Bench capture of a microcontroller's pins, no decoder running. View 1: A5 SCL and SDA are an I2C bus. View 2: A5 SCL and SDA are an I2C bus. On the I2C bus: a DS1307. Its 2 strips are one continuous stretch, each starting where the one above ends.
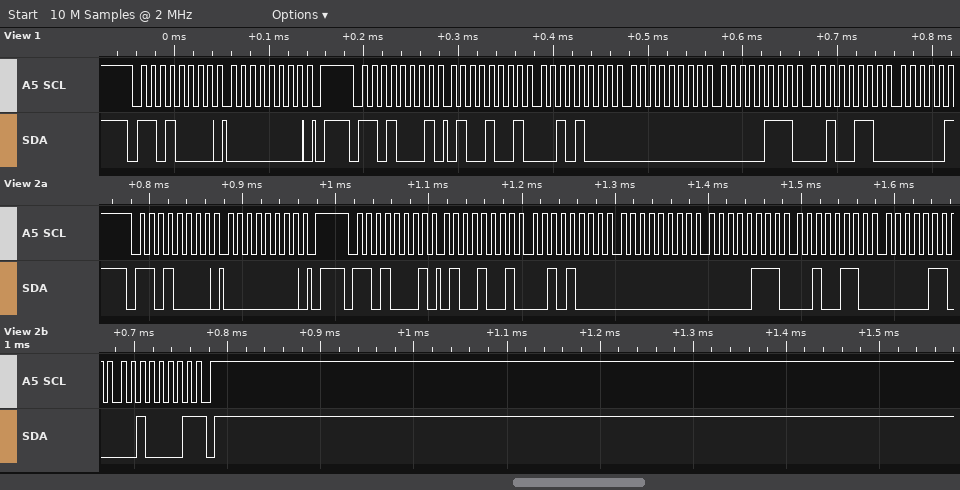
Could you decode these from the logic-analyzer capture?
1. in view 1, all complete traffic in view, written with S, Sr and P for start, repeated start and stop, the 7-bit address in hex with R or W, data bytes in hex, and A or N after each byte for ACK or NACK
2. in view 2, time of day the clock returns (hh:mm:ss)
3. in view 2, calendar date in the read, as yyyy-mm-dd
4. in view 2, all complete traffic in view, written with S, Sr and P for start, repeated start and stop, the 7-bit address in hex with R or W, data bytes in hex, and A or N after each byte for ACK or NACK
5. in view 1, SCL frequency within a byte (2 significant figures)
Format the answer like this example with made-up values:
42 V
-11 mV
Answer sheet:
S 68W A 00 A P S 68R A 49 A 28 A 00 A 07 A 26 A
00:28:49
2021-06-26
S 68W A 00 A P S 68R A 49 A 28 A 00 A 07 A 26 A 06 A 21 N P
100 kHz
